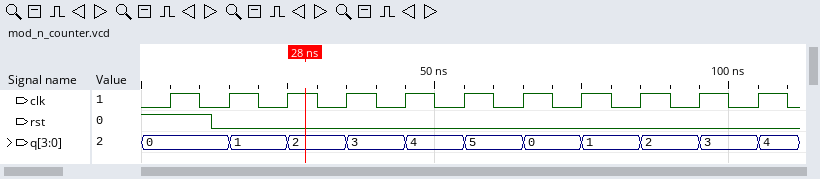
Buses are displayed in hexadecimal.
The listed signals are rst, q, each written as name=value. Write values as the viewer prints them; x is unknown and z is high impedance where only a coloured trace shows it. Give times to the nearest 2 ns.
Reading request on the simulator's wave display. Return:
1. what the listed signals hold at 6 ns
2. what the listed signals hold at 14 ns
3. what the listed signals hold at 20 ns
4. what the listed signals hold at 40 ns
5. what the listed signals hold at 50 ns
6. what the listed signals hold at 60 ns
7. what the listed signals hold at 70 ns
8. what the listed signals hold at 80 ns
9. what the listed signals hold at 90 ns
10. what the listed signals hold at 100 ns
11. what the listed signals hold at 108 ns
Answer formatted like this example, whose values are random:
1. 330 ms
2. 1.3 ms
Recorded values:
1. rst=1, q=0
2. rst=0, q=0
3. rst=0, q=1
4. rst=0, q=3
5. rst=0, q=4
6. rst=0, q=5
7. rst=0, q=0
8. rst=0, q=1
9. rst=0, q=2
10. rst=0, q=3
11. rst=0, q=4
